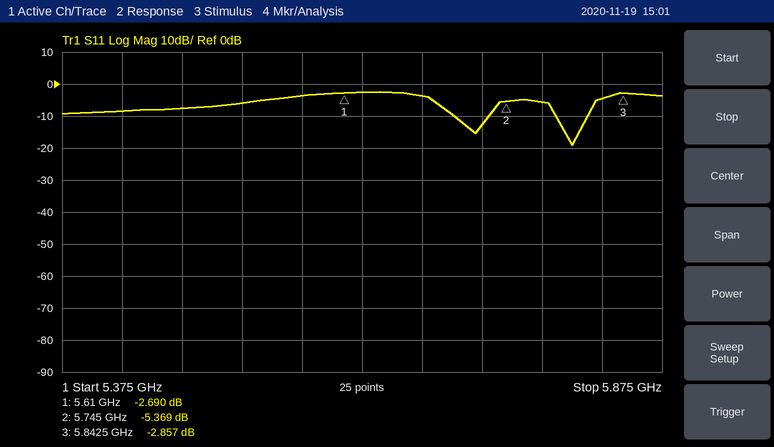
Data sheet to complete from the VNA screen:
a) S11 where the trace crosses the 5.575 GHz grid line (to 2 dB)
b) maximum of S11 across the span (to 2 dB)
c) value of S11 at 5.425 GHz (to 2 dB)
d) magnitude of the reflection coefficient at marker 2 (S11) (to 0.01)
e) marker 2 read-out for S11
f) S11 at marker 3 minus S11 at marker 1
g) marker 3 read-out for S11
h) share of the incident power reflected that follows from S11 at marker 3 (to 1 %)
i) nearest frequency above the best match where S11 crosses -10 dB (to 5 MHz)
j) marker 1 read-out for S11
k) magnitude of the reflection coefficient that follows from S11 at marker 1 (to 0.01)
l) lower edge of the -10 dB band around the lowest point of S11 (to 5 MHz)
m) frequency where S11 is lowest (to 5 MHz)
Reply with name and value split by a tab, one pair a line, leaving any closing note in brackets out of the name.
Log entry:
S11 where the trace crosses the 5.575 GHz grid line	-4 dB
maximum of S11 across the span	-2 dB
value of S11 at 5.425 GHz	-8 dB
magnitude of the reflection coefficient at marker 2 (S11)	0.54
marker 2 read-out for S11	-5.369 dB
S11 at marker 3 minus S11 at marker 1	-0.167 dB
marker 3 read-out for S11	-2.857 dB
share of the incident power reflected that follows from S11 at marker 3	52 %
nearest frequency above the best match where S11 crosses -10 dB	5.815 GHz
marker 1 read-out for S11	-2.690 dB
magnitude of the reflection coefficient that follows from S11 at marker 1	0.73
lower edge of the -10 dB band around the lowest point of S11	5.785 GHz
frequency where S11 is lowest	5.800 GHz
